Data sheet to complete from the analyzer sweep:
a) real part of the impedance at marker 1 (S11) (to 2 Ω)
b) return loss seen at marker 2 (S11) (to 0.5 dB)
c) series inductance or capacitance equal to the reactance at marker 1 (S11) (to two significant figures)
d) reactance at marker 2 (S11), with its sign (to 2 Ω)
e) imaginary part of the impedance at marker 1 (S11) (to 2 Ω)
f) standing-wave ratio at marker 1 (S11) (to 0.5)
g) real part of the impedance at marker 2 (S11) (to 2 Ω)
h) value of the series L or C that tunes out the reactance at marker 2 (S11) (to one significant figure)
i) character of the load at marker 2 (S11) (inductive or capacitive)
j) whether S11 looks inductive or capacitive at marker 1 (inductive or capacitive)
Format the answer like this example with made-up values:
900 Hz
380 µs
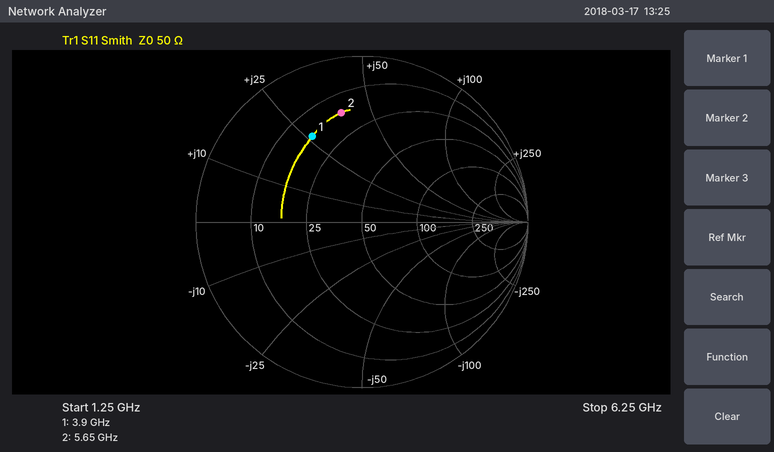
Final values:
16 Ω
3.5 dB
1.1 nH
+38 Ω
+26 Ω
4.0
16 Ω
700 fF
inductive
inductive
